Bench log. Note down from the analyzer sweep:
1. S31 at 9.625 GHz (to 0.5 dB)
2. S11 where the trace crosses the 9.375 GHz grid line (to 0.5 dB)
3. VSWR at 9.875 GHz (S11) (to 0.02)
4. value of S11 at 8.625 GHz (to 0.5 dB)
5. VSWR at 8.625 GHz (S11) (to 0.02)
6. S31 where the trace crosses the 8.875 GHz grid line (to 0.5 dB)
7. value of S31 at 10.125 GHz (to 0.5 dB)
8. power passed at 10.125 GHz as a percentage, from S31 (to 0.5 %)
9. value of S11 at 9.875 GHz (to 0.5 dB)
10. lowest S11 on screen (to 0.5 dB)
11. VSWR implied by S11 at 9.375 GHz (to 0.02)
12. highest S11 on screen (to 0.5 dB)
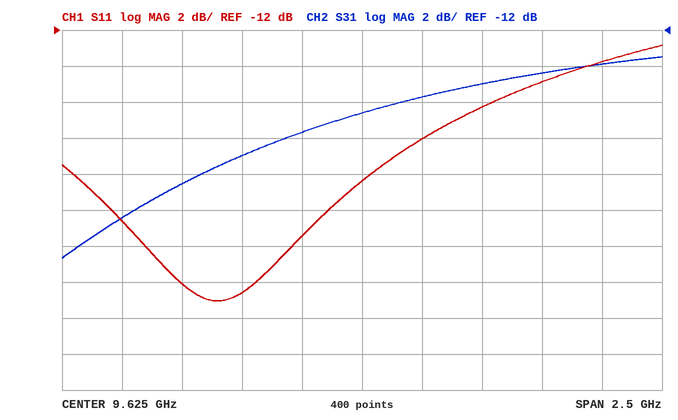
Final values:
-16.5 dB
-23.5 dB
1.28
-22.5 dB
1.16
-20.5 dB
-15.0 dB
3.0 %
-18.0 dB
-27.0 dB
1.14
-13.0 dB
